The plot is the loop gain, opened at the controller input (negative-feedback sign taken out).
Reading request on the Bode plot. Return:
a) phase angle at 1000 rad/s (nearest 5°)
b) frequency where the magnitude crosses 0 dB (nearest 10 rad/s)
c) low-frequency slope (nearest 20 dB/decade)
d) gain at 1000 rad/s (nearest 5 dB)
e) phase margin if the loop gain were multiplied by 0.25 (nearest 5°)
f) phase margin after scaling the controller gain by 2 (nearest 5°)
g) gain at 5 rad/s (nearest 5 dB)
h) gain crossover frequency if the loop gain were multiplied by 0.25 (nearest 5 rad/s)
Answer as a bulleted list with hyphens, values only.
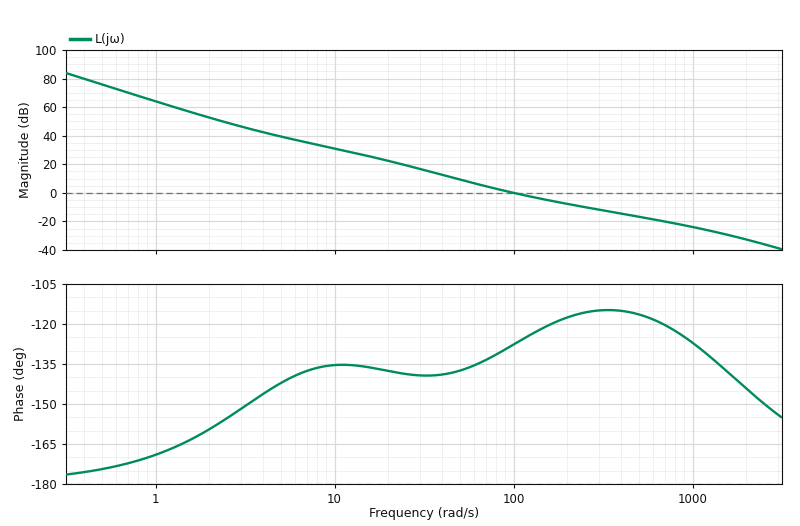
- -125°
- 100 rad/s
- -40 dB/decade
- -25 dB
- 40°
- 60°
- 40 dB
- 40 rad/s
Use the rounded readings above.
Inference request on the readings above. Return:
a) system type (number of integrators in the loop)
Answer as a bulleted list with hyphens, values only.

- 2
